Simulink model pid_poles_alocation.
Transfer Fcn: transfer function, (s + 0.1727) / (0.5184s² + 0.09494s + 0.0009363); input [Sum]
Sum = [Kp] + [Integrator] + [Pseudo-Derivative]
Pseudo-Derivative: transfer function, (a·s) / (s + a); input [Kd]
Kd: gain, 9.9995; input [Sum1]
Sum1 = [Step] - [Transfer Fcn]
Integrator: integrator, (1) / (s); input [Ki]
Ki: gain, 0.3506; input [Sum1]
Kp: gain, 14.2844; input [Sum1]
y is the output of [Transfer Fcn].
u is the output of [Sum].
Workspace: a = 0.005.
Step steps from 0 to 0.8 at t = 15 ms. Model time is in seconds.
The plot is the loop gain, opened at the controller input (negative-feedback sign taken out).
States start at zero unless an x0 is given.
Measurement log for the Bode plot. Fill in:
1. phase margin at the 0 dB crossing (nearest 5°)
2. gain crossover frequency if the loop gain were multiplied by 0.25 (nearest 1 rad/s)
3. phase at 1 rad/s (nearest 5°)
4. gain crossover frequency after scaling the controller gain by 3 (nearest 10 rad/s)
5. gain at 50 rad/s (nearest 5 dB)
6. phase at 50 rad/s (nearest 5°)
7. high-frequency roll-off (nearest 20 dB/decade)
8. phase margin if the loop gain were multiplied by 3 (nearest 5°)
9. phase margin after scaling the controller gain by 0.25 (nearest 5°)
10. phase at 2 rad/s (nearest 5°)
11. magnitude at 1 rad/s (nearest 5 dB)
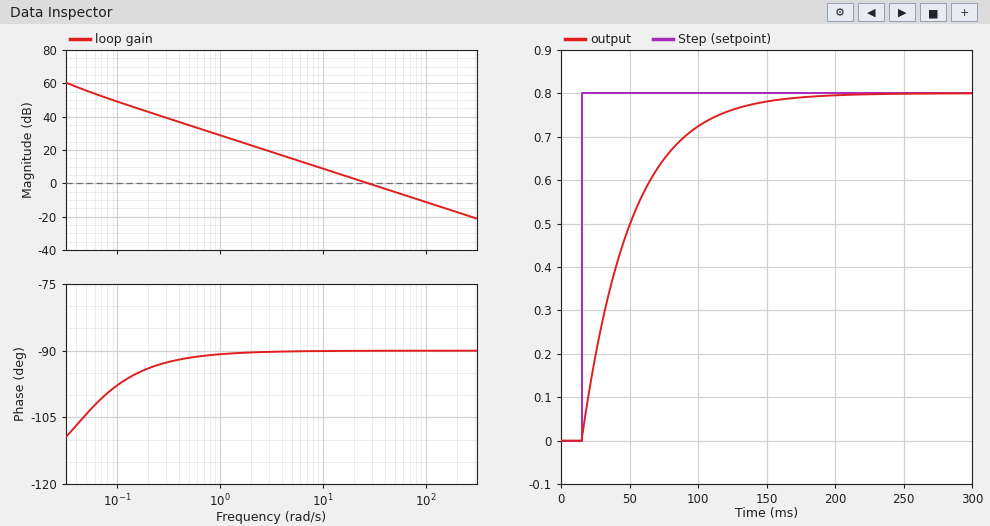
90°
7 rad/s
-90°
80 rad/s
-5 dB
-90°
-20 dB/decade
90°
90°
-90°
30 dB
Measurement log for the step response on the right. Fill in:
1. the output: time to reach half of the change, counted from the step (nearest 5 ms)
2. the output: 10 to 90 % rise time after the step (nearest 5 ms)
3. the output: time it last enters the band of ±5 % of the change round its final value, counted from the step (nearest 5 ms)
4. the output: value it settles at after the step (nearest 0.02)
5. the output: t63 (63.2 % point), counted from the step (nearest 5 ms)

25 ms
80 ms
110 ms
0.80
35 ms
